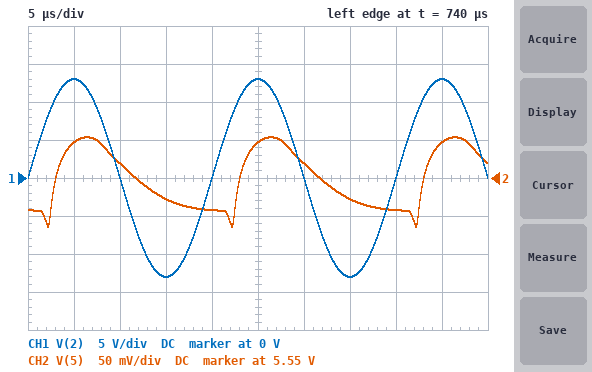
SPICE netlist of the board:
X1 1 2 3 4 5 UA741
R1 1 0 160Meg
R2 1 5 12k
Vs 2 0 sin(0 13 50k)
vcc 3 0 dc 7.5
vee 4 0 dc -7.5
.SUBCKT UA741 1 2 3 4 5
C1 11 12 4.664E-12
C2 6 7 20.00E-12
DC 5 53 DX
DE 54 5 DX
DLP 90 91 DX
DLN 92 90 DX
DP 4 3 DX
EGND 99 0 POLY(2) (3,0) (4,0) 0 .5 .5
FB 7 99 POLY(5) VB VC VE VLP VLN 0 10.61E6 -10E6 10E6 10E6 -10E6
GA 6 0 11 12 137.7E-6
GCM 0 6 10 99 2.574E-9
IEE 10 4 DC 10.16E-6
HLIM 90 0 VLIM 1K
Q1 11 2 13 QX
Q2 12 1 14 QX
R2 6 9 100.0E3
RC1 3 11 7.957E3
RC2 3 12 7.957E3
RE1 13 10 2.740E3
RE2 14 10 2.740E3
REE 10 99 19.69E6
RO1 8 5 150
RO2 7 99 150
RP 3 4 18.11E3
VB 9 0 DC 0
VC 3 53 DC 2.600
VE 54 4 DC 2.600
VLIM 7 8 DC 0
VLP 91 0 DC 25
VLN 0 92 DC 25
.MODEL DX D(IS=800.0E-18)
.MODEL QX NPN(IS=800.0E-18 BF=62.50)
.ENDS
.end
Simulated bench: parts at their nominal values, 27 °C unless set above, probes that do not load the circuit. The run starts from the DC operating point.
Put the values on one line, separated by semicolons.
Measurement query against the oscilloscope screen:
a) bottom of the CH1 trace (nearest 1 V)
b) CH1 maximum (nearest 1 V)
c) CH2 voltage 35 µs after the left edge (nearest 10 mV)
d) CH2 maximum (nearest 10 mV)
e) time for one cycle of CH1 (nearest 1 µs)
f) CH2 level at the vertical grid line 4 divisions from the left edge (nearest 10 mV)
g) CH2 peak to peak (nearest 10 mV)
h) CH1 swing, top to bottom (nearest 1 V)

-13 V; 13 V; 5.52 V; 5.60 V; 20 µs; 5.51 V; 120 mV; 26 V
